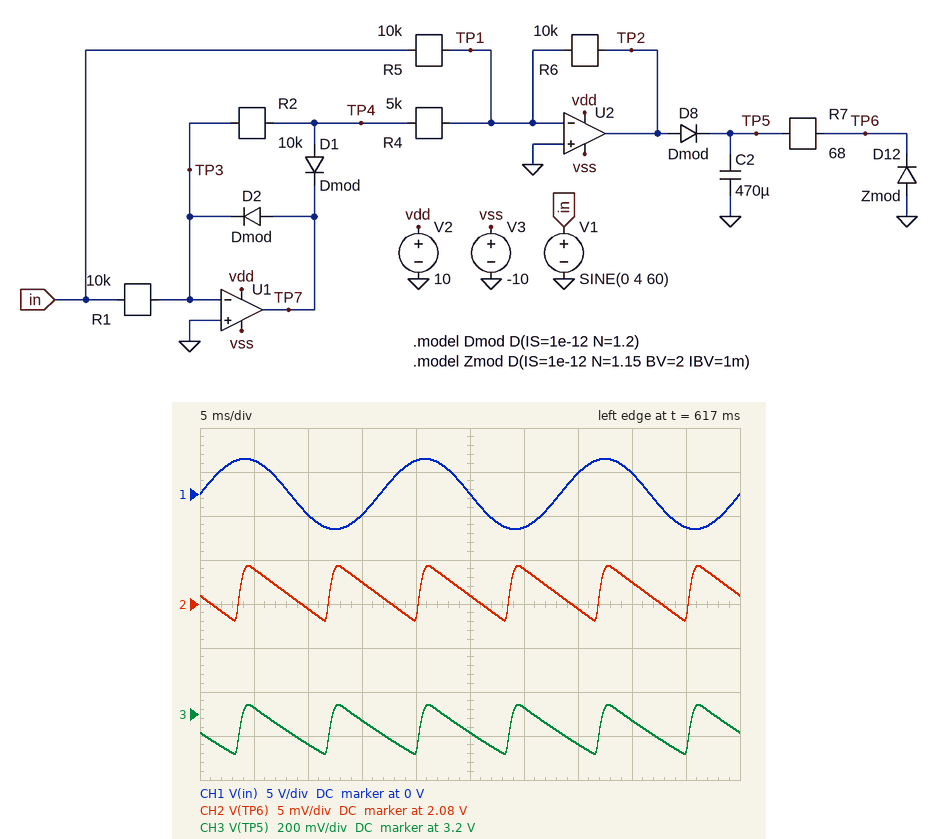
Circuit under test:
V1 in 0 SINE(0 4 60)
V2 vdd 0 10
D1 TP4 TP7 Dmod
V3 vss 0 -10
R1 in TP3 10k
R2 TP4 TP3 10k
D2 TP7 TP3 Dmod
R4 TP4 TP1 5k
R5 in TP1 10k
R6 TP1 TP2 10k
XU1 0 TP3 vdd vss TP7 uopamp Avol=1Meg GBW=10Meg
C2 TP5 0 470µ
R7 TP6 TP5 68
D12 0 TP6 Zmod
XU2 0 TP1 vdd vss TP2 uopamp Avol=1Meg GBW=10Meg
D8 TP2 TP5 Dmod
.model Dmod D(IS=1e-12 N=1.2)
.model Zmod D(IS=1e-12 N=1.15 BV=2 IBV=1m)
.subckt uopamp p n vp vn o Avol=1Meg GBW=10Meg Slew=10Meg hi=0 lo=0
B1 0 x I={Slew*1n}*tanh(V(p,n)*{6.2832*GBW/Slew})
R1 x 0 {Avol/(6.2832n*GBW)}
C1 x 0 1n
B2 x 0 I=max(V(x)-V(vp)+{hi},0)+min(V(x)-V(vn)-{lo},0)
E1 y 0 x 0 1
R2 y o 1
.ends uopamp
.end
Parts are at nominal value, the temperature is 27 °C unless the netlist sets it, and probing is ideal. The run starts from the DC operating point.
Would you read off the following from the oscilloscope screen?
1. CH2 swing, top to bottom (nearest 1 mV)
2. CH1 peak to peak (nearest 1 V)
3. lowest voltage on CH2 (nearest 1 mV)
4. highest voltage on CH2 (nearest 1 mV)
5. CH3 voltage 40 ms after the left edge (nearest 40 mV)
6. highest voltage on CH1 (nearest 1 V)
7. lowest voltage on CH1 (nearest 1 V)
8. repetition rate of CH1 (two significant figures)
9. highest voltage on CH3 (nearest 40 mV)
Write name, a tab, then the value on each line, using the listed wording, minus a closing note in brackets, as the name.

CH2 swing, top to bottom	6 mV
CH1 peak to peak	8 V
lowest voltage on CH2	2.078 V
highest voltage on CH2	2.084 V
CH3 voltage 40 ms after the left edge	3.16 V
highest voltage on CH1	4 V
lowest voltage on CH1	-4 V
repetition rate of CH1	60 Hz
highest voltage on CH3	3.24 V
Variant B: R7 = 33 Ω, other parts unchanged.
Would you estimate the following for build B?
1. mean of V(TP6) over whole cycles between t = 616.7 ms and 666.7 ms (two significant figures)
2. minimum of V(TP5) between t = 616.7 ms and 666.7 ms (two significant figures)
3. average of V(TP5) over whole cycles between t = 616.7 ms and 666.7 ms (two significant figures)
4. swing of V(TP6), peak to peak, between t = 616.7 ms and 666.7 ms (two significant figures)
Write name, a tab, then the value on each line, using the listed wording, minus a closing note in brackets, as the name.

mean of V(TP6) over whole cycles between t = 616.7 ms and 666.7 ms	2.1 V
minimum of V(TP5) between t = 616.7 ms and 666.7 ms	2.8 V
average of V(TP5) over whole cycles between t = 616.7 ms and 666.7 ms	3.0 V
swing of V(TP6), peak to peak, between t = 616.7 ms and 666.7 ms	12 mV
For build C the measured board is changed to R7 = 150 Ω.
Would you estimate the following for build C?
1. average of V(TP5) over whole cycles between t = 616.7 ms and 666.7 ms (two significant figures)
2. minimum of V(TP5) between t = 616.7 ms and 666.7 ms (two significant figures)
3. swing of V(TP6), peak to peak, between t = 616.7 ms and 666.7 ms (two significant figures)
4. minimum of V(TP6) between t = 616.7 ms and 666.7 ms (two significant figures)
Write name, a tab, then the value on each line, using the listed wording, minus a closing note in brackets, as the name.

average of V(TP5) over whole cycles between t = 616.7 ms and 666.7 ms	3.2 V
minimum of V(TP5) between t = 616.7 ms and 666.7 ms	3.1 V
swing of V(TP6), peak to peak, between t = 616.7 ms and 666.7 ms	2.9 mV
minimum of V(TP6) between t = 616.7 ms and 666.7 ms	2.1 V
